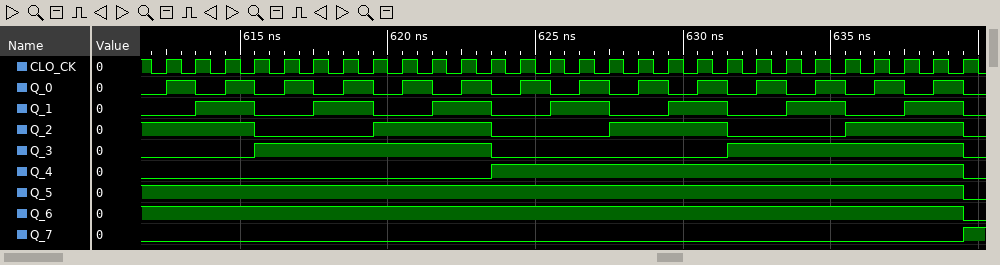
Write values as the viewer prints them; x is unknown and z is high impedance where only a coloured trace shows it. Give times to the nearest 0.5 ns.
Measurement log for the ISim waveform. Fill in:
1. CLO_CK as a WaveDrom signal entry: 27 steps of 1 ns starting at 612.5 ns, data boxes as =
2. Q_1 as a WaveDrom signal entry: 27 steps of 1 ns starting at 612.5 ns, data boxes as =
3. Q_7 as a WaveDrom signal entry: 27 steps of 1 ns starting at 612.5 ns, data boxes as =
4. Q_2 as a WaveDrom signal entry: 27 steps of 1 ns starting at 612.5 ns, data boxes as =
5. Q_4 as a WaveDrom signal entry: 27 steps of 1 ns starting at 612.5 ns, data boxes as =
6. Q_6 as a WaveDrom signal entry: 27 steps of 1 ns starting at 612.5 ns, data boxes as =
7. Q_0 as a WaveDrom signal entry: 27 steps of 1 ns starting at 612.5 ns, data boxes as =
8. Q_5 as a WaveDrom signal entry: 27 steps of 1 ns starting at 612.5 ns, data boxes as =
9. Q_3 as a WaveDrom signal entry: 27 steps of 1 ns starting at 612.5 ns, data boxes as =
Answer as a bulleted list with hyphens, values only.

- {name: 'CLO_CK', wave: 'p..........................'}
- {name: 'Q_1', wave: '01.0.1.0.1.0.1.0.1.0.1.0.1.'}
- {name: 'Q_7', wave: '0..........................'}
- {name: 'Q_2', wave: '1..0...1...0...1...0...1...'}
- {name: 'Q_4', wave: '0..........1...............'}
- {name: 'Q_6', wave: '1..........................'}
- {name: 'Q_0', wave: '101010101010101010101010101'}
- {name: 'Q_5', wave: '1..........................'}
- {name: 'Q_3', wave: '0..1.......0.......1.......'}
